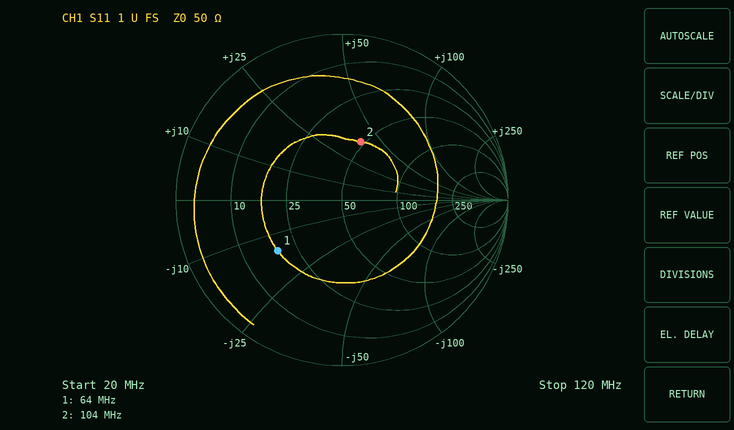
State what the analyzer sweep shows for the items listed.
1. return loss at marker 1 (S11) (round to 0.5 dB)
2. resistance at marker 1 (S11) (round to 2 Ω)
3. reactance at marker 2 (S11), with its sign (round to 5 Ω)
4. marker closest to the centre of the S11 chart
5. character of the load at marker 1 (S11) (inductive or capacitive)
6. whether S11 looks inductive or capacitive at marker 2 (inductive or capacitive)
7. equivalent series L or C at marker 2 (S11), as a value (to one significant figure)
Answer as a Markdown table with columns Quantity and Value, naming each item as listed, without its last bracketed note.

| Quantity | Value |
|---|---|
| return loss at marker 1 (S11) | 6.0 dB |
| resistance at marker 1 (S11) | 18 Ω |
| reactance at marker 2 (S11), with its sign | +40 Ω |
| marker closest to the centre of the S11 chart | marker 2 |
| character of the load at marker 1 (S11) | capacitive |
| whether S11 looks inductive or capacitive at marker 2 | inductive |
| equivalent series L or C at marker 2 (S11), as a value | 60 nH |
